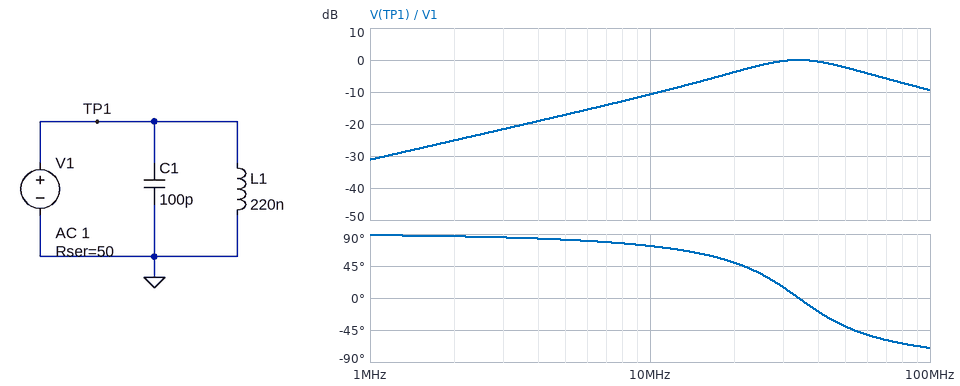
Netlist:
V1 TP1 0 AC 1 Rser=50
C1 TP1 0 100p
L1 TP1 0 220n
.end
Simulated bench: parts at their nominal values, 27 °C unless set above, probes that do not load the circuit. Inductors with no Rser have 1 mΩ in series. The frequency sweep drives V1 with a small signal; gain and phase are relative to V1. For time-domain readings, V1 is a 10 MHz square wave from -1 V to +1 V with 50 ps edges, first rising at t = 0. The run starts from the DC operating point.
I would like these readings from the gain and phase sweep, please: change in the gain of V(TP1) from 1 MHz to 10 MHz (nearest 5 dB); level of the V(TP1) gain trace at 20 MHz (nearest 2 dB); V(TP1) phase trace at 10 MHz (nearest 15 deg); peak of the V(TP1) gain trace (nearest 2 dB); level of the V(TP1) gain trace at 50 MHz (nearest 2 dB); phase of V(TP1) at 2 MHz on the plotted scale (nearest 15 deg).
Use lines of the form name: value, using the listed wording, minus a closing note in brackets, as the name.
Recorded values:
change in the gain of V(TP1) from 1 MHz to 10 MHz: 20 dB
level of the V(TP1) gain trace at 20 MHz: -4 dB
V(TP1) phase trace at 10 MHz: 75 deg
peak of the V(TP1) gain trace: 0 dB
level of the V(TP1) gain trace at 50 MHz: -2 dB
phase of V(TP1) at 2 MHz on the plotted scale: 90 deg
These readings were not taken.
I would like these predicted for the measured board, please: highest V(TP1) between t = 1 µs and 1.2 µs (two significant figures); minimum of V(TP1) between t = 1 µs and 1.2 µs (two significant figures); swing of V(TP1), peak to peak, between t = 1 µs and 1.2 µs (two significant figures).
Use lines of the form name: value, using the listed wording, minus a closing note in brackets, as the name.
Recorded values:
highest V(TP1) between t = 1 µs and 1.2 µs: 1.1 V
minimum of V(TP1) between t = 1 µs and 1.2 µs: -1.1 V
swing of V(TP1), peak to peak, between t = 1 µs and 1.2 µs: 2.1 V
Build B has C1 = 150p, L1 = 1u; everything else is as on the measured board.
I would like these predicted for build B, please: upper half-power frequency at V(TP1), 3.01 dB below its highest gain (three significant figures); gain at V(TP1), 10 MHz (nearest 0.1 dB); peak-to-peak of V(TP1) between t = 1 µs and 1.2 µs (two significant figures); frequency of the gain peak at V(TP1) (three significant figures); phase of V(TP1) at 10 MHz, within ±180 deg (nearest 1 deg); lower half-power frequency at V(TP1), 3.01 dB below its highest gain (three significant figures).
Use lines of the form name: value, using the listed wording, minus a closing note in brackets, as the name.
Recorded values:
upper half-power frequency at V(TP1), 3.01 dB below its highest gain: 27.4 MHz
gain at V(TP1), 10 MHz: -0.4 dB
peak-to-peak of V(TP1) between t = 1 µs and 1.2 µs: 2.7 V
frequency of the gain peak at V(TP1): 13.0 MHz
phase of V(TP1) at 10 MHz, within ±180 deg: 18 deg
lower half-power frequency at V(TP1), 3.01 dB below its highest gain: 6.17 MHz
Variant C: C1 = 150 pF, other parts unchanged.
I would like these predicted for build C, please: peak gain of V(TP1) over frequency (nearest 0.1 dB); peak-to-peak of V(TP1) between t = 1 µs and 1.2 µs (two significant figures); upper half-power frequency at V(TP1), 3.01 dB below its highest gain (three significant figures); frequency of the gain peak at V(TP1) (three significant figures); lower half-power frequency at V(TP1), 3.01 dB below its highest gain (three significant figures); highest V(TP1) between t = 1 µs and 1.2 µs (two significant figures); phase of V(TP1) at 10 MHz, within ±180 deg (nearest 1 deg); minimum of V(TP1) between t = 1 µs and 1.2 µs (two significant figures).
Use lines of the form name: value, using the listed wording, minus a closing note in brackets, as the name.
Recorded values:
peak gain of V(TP1) over frequency: 0 dB
peak-to-peak of V(TP1) between t = 1 µs and 1.2 µs: 1.9 V
upper half-power frequency at V(TP1), 3.01 dB below its highest gain: 40.3 MHz
frequency of the gain peak at V(TP1): 27.7 MHz
lower half-power frequency at V(TP1), 3.01 dB below its highest gain: 19.1 MHz
highest V(TP1) between t = 1 µs and 1.2 µs: 930 mV
phase of V(TP1) at 10 MHz, within ±180 deg: 72 deg
minimum of V(TP1) between t = 1 µs and 1.2 µs: -930 mV
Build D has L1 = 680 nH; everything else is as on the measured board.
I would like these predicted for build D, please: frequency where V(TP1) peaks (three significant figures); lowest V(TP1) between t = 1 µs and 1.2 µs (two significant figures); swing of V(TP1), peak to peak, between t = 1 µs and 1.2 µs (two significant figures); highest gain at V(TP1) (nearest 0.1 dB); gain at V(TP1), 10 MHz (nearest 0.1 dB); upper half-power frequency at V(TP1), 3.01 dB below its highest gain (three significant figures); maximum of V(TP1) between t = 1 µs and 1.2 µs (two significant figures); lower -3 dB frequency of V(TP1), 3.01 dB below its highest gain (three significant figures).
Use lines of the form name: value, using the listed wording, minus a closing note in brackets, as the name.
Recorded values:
frequency where V(TP1) peaks: 19.3 MHz
lowest V(TP1) between t = 1 µs and 1.2 µs: -1.4 V
swing of V(TP1), peak to peak, between t = 1 µs and 1.2 µs: 2.8 V
highest gain at V(TP1): 0 dB
gain at V(TP1), 10 MHz: -2.4 dB
upper half-power frequency at V(TP1), 3.01 dB below its highest gain: 40.9 MHz
maximum of V(TP1) between t = 1 µs and 1.2 µs: 1.4 V
lower -3 dB frequency of V(TP1), 3.01 dB below its highest gain: 9.10 MHz
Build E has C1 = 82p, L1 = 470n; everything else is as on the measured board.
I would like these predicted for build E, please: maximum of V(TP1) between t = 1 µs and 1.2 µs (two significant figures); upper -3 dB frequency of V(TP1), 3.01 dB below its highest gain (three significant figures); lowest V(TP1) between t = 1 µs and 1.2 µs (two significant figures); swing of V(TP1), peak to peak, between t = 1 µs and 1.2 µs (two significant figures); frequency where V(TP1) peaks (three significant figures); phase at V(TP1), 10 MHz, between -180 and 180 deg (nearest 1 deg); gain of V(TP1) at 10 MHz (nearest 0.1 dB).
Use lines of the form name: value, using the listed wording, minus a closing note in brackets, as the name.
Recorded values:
maximum of V(TP1) between t = 1 µs and 1.2 µs: 1.3 V
upper -3 dB frequency of V(TP1), 3.01 dB below its highest gain: 51.6 MHz
lowest V(TP1) between t = 1 µs and 1.2 µs: -1.3 V
swing of V(TP1), peak to peak, between t = 1 µs and 1.2 µs: 2.7 V
frequency where V(TP1) peaks: 25.6 MHz
phase at V(TP1), 10 MHz, between -180 and 180 deg: 55 deg
gain of V(TP1) at 10 MHz: -4.9 dB
